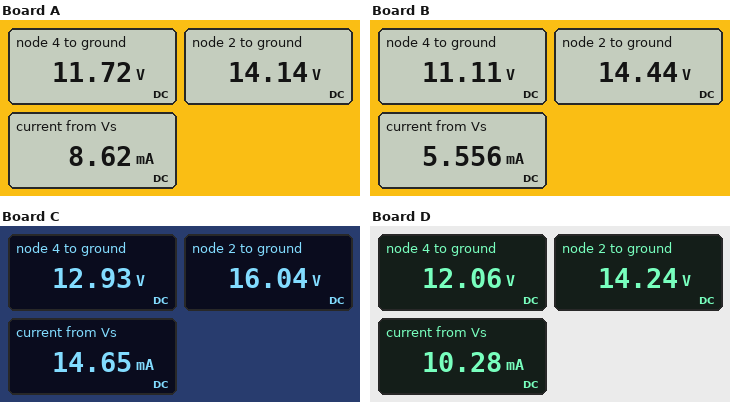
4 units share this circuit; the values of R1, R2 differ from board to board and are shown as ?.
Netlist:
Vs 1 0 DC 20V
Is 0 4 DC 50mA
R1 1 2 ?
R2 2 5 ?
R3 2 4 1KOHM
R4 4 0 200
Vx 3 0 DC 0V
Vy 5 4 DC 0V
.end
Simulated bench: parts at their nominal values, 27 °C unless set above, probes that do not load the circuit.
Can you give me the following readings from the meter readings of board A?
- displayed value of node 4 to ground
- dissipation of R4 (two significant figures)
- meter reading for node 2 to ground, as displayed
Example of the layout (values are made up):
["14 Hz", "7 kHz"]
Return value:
["11.72 V", "690 mW", "14.14 V"]
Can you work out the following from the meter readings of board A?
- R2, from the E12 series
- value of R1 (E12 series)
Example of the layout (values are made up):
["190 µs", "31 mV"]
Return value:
["390 Ω", "680 Ω"]
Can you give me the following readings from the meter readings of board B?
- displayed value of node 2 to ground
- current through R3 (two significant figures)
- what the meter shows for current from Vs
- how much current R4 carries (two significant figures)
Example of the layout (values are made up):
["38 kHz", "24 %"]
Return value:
["14.44 V", "3.3 mA", "5.556 mA", "56 mA"]
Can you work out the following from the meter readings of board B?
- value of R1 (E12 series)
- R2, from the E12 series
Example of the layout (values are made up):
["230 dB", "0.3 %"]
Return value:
["1 kΩ", "1.5 kΩ"]
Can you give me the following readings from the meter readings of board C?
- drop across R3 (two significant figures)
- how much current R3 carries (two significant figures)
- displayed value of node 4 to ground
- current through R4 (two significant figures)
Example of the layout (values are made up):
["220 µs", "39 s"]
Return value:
["3.1 V", "3.1 mA", "12.93 V", "65 mA"]
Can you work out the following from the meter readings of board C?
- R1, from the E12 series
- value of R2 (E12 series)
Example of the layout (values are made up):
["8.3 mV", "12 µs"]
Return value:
["270 Ω", "270 Ω"]
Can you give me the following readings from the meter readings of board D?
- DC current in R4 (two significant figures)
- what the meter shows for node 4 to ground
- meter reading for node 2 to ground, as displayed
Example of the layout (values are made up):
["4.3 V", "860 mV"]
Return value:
["60 mA", "12.06 V", "14.24 V"]
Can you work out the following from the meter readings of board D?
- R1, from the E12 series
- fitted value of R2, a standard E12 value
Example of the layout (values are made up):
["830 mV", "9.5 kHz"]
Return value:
["560 Ω", "270 Ω"]
